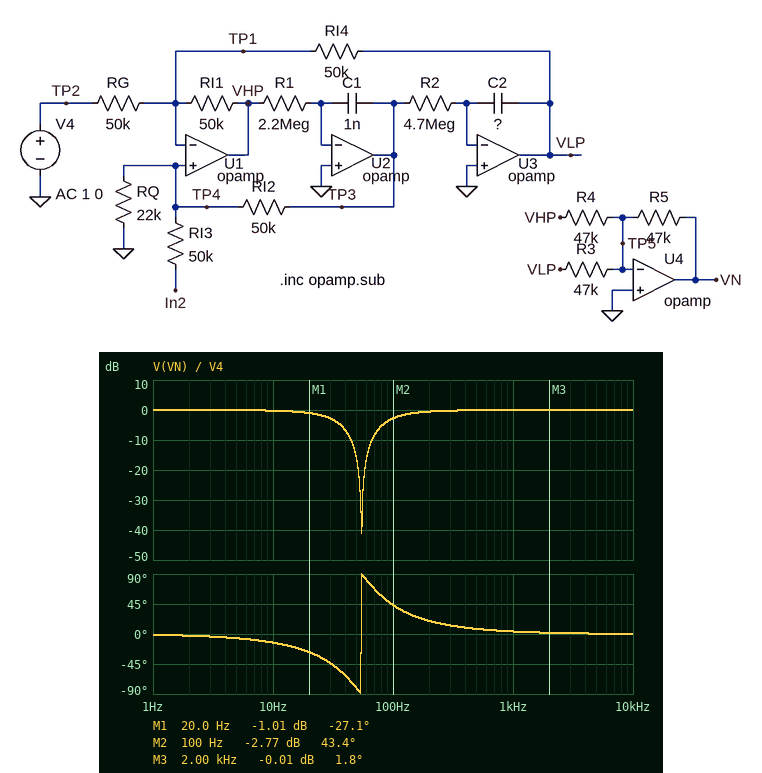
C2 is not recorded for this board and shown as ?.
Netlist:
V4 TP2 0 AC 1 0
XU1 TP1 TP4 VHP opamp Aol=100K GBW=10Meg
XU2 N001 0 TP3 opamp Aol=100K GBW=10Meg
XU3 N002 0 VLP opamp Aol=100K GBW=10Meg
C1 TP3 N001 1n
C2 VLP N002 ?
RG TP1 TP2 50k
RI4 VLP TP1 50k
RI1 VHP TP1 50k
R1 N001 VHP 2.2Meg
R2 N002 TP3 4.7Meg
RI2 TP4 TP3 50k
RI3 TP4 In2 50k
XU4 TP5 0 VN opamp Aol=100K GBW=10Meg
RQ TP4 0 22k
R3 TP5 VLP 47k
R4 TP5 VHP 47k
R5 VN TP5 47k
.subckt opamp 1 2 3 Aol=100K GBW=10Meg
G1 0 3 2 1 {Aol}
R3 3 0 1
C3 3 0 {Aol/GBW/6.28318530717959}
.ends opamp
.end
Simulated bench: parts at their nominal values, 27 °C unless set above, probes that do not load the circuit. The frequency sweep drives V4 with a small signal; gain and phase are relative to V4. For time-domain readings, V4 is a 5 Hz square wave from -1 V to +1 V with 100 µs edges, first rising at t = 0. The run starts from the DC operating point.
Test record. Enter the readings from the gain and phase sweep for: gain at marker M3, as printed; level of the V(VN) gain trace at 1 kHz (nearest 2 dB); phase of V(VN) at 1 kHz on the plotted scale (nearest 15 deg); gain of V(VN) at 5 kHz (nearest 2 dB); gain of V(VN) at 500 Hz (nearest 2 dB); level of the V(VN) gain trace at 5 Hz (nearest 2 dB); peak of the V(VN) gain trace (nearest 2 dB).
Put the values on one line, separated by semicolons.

-0.01 dB; 0 dB; 0 deg; 0 dB; 0 dB; 0 dB; 0 dB
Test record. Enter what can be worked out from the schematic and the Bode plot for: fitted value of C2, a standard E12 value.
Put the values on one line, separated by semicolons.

820 pF
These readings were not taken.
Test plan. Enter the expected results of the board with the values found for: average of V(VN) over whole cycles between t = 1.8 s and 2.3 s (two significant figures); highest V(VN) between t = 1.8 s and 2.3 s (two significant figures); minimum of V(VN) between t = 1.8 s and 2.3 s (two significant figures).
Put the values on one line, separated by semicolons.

180 mV; 1.1 V; -1.1 V
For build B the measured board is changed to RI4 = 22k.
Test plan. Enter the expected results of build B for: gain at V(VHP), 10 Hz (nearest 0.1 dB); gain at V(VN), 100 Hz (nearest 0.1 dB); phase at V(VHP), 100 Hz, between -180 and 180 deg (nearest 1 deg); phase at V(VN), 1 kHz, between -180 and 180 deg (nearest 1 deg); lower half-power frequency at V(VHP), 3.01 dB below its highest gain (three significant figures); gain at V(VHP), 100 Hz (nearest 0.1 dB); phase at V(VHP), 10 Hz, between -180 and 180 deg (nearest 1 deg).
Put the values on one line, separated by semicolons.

-36.6 dB; -3.1 dB; -109 deg; 5 deg; 72.8 Hz; 0 dB; -8 deg
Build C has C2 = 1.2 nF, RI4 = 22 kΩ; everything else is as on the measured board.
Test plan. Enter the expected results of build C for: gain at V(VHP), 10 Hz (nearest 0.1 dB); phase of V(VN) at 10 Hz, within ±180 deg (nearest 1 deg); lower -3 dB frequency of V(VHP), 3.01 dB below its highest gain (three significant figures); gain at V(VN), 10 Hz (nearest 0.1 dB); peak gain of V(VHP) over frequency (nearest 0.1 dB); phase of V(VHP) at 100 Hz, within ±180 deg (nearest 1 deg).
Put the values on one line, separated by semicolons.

-33.3 dB; -12 deg; 66.9 Hz; -7.6 dB; 0 dB; -120 deg
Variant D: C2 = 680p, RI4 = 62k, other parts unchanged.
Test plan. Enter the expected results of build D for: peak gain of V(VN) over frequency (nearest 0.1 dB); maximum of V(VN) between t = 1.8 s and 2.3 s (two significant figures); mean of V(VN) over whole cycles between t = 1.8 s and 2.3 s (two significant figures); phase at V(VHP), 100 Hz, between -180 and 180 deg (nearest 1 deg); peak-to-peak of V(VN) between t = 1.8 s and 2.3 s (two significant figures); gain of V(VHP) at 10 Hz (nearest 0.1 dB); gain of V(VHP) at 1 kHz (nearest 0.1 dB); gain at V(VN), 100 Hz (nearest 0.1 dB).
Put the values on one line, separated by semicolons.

1.9 dB; 1.4 V; 230 mV; -139 deg; 2.8 V; -29.2 dB; 0 dB; -3.4 dB
